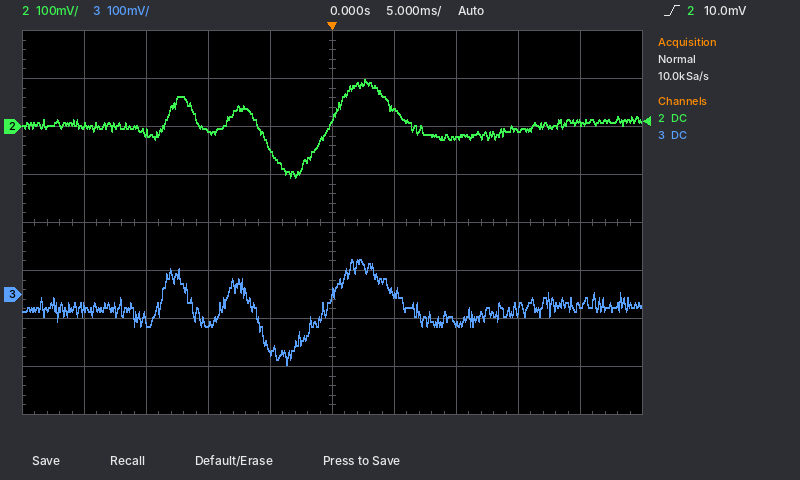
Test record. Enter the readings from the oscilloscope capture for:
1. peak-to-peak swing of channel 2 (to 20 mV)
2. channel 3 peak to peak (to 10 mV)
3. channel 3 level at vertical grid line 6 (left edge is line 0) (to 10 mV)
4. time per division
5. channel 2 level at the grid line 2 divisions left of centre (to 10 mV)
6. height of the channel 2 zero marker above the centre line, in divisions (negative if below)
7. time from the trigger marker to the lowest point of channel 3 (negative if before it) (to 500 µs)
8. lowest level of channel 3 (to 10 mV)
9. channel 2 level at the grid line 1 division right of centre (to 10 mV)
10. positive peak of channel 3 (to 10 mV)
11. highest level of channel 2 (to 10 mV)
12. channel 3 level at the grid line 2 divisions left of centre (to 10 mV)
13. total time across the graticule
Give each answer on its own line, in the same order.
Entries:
200 mV
220 mV
0 mV
5 ms
-10 mV
+2.0 div
-3.5 ms
-150 mV
40 mV
70 mV
100 mV
-60 mV
50 ms
